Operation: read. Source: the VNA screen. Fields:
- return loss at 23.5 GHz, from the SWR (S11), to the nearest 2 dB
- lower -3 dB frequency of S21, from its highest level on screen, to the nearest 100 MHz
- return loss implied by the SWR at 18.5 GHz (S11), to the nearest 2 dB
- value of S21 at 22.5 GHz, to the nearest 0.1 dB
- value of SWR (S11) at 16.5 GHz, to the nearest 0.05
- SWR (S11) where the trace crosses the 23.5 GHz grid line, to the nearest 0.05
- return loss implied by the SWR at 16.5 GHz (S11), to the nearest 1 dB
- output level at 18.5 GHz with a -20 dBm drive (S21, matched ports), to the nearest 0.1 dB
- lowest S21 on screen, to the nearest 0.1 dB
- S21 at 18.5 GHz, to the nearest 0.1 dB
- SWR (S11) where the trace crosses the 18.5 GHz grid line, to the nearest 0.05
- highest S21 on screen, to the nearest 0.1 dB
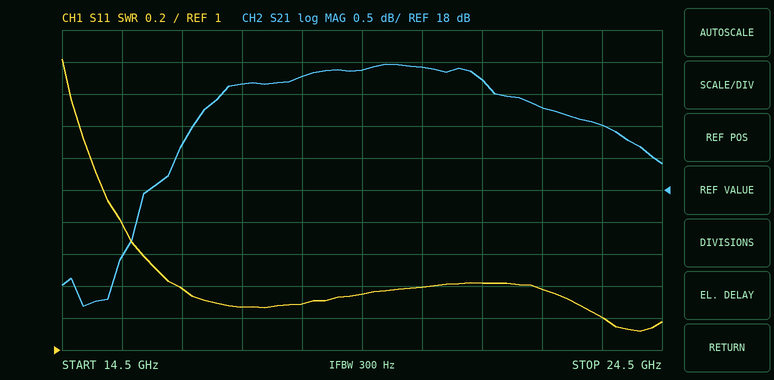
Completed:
20 dB
15.5 GHz
18 dB
19.3 dB
1.40
1.20
16 dB
-0.2 dBm
16.2 dB
19.8 dB
1.30
20.0 dB
